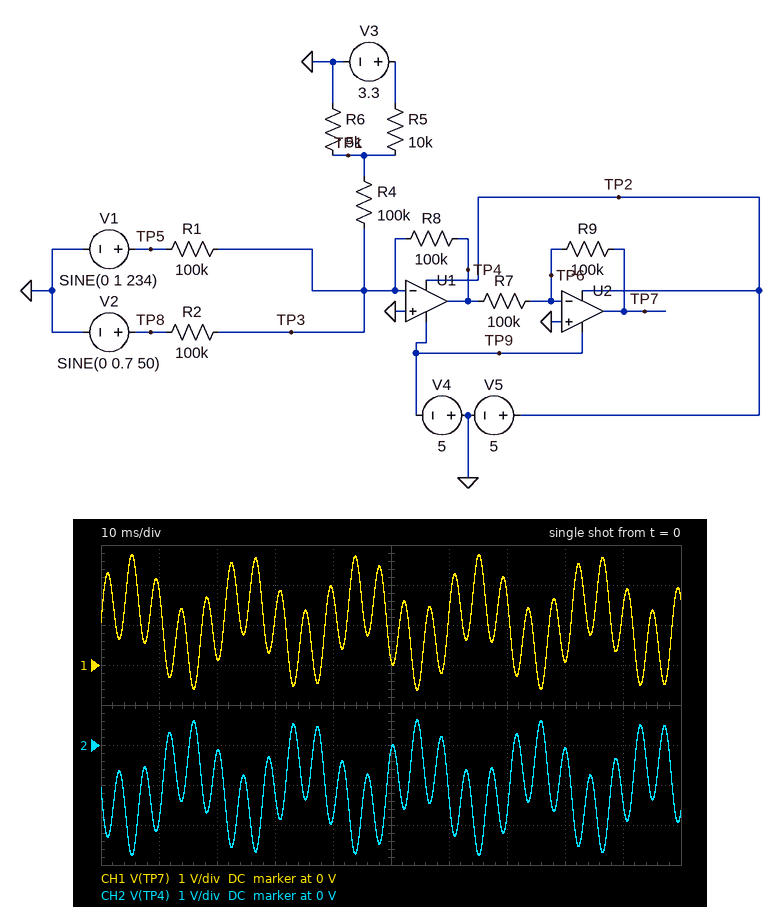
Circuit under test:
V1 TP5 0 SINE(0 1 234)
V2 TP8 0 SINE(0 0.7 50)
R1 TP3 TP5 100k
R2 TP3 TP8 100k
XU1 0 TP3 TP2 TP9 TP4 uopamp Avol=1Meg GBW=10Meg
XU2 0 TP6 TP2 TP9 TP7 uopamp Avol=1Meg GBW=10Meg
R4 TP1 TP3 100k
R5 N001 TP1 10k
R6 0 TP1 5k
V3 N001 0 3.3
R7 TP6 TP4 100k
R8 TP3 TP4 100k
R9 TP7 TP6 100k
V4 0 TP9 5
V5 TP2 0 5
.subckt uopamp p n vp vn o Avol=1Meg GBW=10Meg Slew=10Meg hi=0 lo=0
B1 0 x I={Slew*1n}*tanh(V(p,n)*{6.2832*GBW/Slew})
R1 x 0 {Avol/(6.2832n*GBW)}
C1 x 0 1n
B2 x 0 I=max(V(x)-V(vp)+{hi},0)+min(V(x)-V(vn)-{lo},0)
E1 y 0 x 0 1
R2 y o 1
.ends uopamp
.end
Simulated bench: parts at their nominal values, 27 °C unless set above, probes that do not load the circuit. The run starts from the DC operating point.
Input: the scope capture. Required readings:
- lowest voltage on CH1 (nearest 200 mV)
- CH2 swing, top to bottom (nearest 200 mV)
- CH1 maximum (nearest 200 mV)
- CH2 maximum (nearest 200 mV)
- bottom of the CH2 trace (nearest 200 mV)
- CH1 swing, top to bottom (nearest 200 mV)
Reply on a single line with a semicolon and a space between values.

-600 mV; 3.4 V; 2.8 V; 600 mV; -2.8 V; 3.4 V
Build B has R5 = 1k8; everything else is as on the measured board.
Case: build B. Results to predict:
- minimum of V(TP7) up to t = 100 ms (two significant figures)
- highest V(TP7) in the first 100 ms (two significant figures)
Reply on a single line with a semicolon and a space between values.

700 mV; 4.1 V
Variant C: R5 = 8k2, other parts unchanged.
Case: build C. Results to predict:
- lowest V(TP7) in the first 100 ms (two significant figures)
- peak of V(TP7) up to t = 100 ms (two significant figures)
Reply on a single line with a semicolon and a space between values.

-480 mV; 2.9 V
